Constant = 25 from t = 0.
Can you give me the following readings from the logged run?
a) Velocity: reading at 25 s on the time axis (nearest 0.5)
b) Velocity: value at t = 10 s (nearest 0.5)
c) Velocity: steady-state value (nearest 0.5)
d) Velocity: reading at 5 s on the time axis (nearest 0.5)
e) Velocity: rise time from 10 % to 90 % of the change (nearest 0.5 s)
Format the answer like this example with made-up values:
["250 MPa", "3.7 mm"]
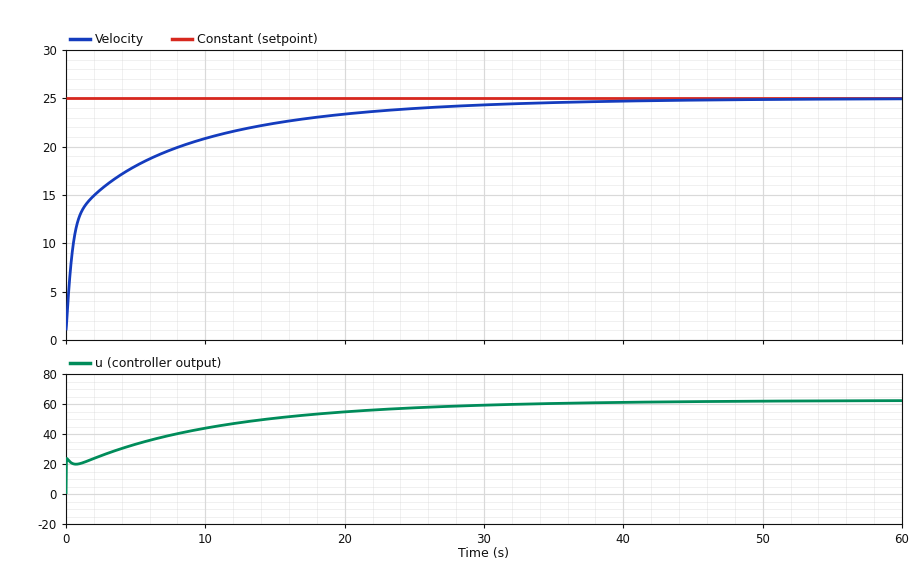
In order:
["24.0", "21.0", "25.0", "18.0", "15.5 s"]
